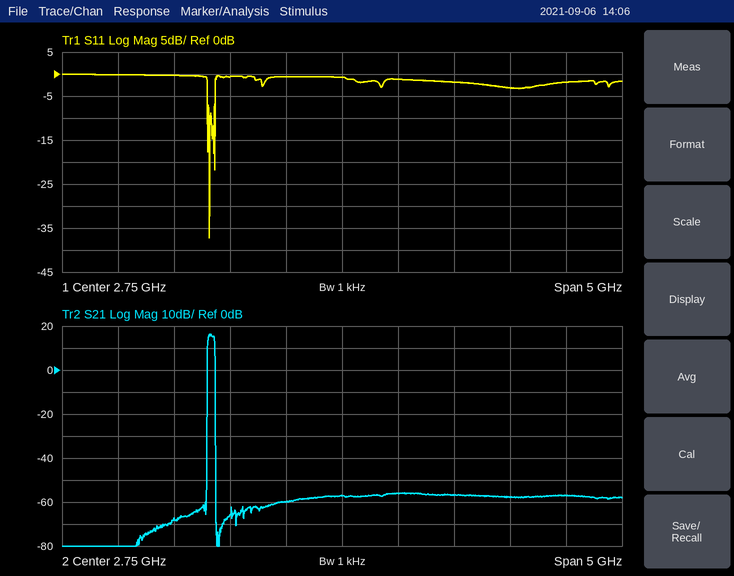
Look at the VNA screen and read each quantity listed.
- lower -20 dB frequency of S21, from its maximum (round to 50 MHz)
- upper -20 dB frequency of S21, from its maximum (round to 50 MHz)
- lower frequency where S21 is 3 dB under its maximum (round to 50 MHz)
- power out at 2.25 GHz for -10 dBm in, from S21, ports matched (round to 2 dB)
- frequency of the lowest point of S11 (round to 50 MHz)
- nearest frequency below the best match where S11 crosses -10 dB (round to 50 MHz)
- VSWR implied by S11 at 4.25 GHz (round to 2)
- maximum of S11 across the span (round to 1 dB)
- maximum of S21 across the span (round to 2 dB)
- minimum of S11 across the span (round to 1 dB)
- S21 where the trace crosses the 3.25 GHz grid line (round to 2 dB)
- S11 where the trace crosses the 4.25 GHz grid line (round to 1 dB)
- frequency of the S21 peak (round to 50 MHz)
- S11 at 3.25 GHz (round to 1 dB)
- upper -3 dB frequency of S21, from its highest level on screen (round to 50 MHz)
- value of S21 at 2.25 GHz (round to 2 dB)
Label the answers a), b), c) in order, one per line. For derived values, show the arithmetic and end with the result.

a) 1.55 GHz
b) 1.60 GHz
c) 1.55 GHz
d) -10 dBm + (-60 dB) = -70 dBm
e) 1.55 GHz
f) 1.55 GHz
g) |Γ| = 10^(-3/20) = 0.7079; VSWR = (1 + 0.7079)/(1 − 0.7079) ≈ 6
h) 0 dB
i) 16 dB
j) -37 dB
k) -56 dB
l) -3 dB
m) 1.55 GHz
n) -1 dB
o) 1.60 GHz
p) -60 dB
